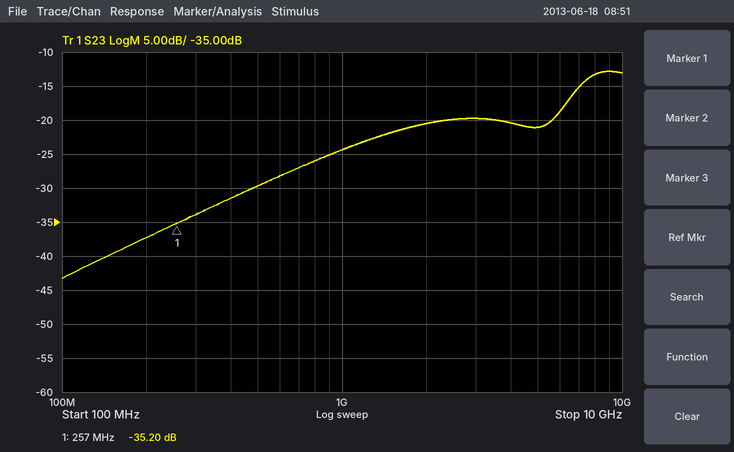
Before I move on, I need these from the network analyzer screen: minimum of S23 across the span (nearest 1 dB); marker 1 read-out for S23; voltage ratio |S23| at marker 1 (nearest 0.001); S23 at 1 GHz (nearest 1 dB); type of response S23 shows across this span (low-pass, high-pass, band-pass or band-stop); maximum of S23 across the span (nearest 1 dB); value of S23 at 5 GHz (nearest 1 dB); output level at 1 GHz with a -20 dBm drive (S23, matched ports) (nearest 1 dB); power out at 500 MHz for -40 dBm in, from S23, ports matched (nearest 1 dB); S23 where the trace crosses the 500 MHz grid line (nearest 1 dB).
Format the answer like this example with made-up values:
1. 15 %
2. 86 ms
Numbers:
1. -43 dB
2. -35.20 dB
3. 0.017
4. -24 dB
5. high-pass
6. -13 dB
7. -21 dB
8. -44 dBm
9. -70 dBm
10. -30 dB
